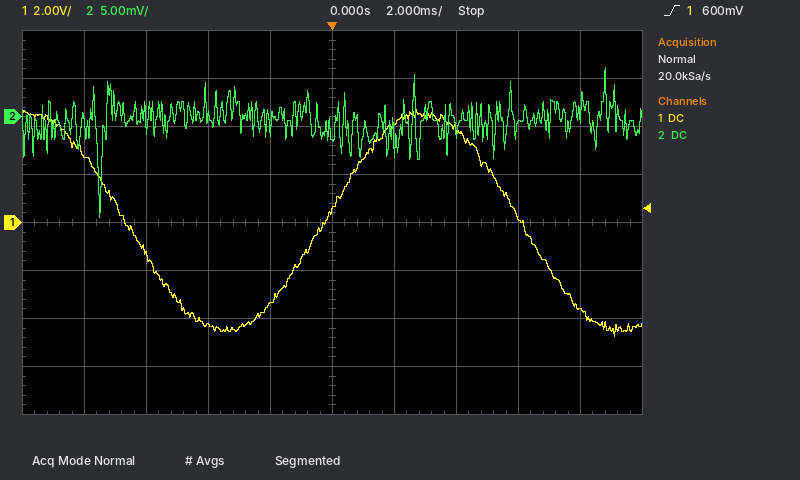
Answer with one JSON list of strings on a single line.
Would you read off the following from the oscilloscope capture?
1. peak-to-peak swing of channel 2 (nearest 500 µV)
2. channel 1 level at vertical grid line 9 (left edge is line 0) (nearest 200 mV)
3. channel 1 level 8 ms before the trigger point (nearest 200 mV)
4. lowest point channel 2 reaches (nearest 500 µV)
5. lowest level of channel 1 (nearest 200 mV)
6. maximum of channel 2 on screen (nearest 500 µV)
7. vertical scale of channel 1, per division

["15.5 mV", "-3.6 V", "2.8 V", "-10.5 mV", "-4.8 V", "5.0 mV", "2 V"]
